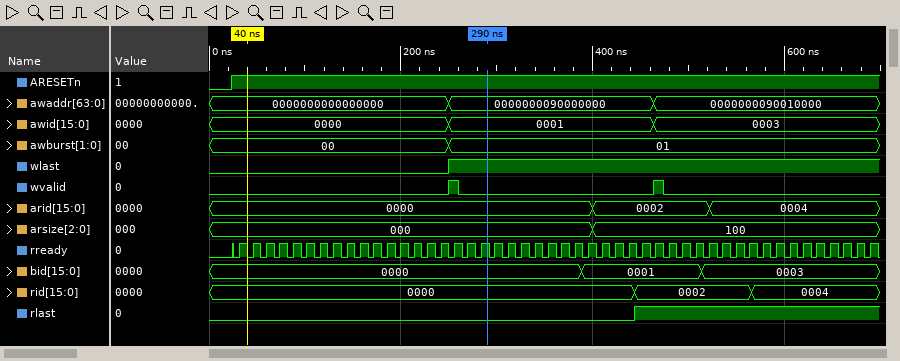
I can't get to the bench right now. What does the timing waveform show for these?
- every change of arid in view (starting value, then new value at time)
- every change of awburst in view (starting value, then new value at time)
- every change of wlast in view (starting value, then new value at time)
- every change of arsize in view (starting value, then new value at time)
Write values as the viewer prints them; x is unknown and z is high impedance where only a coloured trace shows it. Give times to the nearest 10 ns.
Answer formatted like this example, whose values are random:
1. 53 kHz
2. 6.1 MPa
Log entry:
1. 0000, 0002 at 400 ns, 0004 at 520 ns
2. 00, 01 at 250 ns
3. 0, 1 at 250 ns
4. 000, 100 at 400 ns
